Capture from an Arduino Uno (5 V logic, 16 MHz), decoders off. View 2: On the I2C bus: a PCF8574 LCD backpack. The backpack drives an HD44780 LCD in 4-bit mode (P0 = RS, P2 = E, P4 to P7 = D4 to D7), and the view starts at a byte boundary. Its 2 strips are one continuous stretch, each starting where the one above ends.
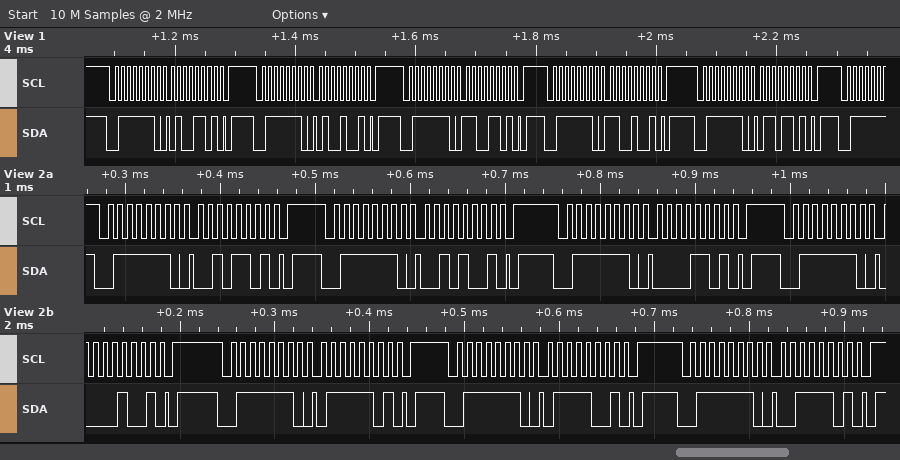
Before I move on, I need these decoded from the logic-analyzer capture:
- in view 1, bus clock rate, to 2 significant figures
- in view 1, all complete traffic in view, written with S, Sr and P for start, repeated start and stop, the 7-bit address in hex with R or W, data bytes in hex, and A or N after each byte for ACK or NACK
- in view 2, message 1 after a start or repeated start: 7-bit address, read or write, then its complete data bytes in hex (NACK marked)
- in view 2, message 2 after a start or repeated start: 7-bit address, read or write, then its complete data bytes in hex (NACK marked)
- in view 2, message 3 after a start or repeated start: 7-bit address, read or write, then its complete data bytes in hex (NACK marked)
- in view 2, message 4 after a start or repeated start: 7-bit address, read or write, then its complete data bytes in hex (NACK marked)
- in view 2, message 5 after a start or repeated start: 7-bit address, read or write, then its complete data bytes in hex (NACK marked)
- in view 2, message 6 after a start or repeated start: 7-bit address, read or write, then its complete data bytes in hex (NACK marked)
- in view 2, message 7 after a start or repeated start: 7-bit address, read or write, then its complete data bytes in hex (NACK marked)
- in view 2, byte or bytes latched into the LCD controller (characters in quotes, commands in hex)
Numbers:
100 kHz
S 3FW A 4D A P S 3FW A 49 A P S 3FW A CD A P S 3FW A C9 A P S 3FW A 6D A P
0x3F write: 2D
0x3F write: 29
0x3F write: 0D
0x3F write: 09
0x3F write: 7D
0x3F write: 79
0x3F write: 3D
' '
